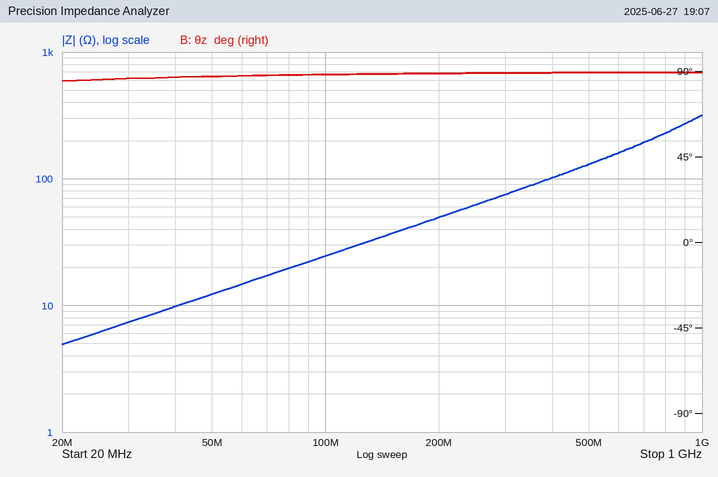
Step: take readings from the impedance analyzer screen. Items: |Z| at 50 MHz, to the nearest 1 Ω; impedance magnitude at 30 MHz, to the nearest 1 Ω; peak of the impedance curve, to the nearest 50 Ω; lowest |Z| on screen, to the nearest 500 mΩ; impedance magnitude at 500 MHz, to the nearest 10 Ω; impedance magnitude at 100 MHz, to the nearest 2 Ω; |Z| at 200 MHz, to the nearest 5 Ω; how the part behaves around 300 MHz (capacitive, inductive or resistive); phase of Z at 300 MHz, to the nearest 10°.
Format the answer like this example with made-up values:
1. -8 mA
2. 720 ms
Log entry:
1. 12 Ω
2. 7 Ω
3. 300 Ω
4. 5.0 Ω
5. 130 Ω
6. 24 Ω
7. 50 Ω
8. inductive
9. 90°
